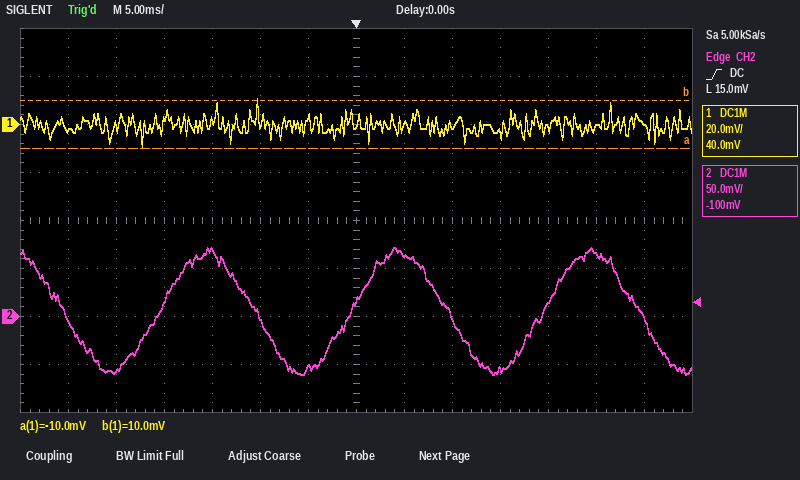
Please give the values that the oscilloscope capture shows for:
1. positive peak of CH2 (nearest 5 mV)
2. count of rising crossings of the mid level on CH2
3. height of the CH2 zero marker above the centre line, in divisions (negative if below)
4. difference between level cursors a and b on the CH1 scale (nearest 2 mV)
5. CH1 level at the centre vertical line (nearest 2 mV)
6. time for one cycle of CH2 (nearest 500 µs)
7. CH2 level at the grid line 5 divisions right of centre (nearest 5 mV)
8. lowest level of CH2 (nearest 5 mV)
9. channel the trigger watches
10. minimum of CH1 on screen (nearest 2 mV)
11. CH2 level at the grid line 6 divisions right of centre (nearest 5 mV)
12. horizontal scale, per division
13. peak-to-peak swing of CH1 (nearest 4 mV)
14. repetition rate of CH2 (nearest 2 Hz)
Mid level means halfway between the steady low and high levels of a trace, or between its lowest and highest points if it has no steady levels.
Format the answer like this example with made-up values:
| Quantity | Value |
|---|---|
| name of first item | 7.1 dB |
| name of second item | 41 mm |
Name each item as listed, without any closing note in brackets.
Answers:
| Quantity | Value |
|---|---|
| positive peak of CH2 | 70 mV |
| count of rising crossings of the mid level on CH2 | 3 |
| height of the CH2 zero marker above the centre line, in divisions | -2.0 div |
| difference between level cursors a and b on the CH1 scale | 20 mV |
| CH1 level at the centre vertical line | 0 mV |
| time for one cycle of CH2 | 20.0 ms |
| CH2 level at the grid line 5 divisions right of centre | 65 mV |
| lowest level of CH2 | -60 mV |
| channel the trigger watches | CH2 |
| minimum of CH1 on screen | -10 mV |
| CH2 level at the grid line 6 divisions right of centre | 0 mV |
| horizontal scale, per division | 5 ms |
| peak-to-peak swing of CH1 | 20 mV |
| repetition rate of CH2 | 50 Hz |
